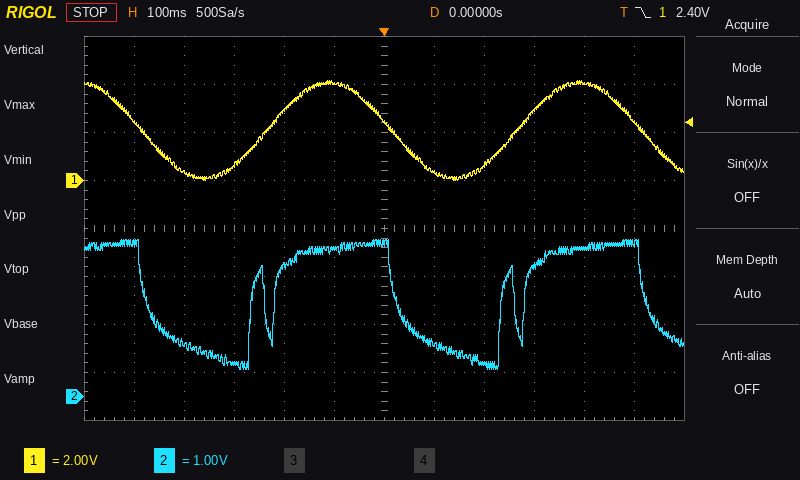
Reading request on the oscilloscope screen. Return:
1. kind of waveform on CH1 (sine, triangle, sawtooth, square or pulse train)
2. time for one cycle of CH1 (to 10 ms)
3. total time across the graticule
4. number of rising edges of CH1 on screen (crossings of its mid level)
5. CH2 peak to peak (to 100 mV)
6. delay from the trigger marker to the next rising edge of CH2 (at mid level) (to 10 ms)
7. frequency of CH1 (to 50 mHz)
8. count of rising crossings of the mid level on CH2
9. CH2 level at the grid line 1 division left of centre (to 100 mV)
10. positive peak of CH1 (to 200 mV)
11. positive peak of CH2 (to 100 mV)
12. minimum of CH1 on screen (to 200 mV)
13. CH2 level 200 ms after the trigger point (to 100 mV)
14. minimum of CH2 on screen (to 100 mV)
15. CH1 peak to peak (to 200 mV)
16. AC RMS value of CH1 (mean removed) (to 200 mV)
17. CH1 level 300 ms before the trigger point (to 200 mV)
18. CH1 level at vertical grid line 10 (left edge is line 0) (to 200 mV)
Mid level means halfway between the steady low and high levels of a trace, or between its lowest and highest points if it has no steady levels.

sine
500 ms
1.2 s
2
2.7 V
230 ms
2.00 Hz
4
3.1 V
4.2 V
3.3 V
0.0 V
700 mV
600 mV
4.2 V
1.4 V
600 mV
4.0 V
